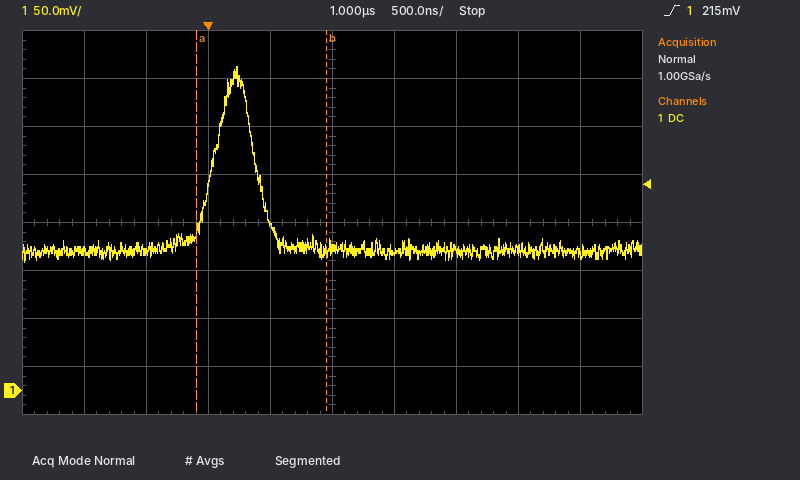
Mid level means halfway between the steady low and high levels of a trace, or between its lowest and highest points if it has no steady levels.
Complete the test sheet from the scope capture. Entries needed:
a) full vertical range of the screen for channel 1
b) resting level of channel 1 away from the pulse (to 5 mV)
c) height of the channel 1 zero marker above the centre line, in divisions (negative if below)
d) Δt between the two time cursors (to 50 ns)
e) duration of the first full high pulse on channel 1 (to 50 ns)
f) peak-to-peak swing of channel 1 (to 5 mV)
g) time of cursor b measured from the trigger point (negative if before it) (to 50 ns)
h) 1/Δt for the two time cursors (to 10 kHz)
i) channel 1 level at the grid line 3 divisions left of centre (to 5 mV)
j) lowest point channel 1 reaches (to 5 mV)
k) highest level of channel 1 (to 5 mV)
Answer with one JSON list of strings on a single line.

["400 mV", "145 mV", "-3.5 div", "1.05 µs", "350 ns", "205 mV", "+950 ns", "950 kHz", "145 mV", "135 mV", "340 mV"]
